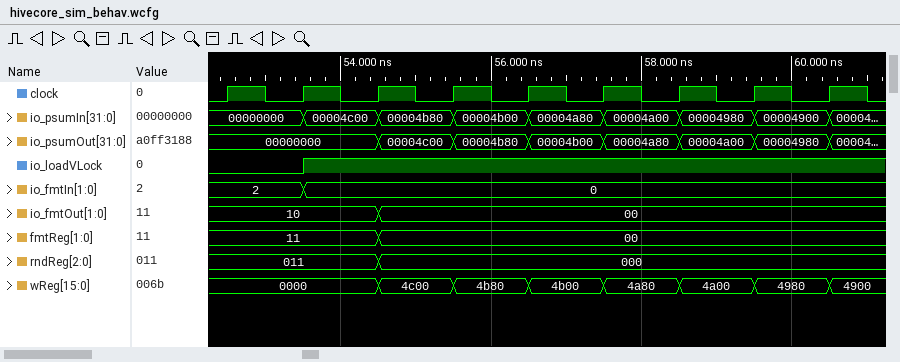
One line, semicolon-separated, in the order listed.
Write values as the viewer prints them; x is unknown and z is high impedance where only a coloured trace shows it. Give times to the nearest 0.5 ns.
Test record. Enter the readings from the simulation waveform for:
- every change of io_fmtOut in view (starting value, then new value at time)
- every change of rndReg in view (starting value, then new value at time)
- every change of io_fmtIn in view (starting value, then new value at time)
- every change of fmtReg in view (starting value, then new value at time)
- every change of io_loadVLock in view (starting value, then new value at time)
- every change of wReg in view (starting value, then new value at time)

10, 00 at 54.5 ns; 011, 000 at 54.5 ns; 2, 0 at 53.5 ns; 11, 00 at 54.5 ns; 0, 1 at 53.5 ns; 0000, 4c00 at 54.5 ns, 4b80 at 55.5 ns, 4b00 at 56.5 ns, 4a80 at 57.5 ns, 4a00 at 58.5 ns, 4980 at 59.5 ns, 4900 at 60.5 ns
